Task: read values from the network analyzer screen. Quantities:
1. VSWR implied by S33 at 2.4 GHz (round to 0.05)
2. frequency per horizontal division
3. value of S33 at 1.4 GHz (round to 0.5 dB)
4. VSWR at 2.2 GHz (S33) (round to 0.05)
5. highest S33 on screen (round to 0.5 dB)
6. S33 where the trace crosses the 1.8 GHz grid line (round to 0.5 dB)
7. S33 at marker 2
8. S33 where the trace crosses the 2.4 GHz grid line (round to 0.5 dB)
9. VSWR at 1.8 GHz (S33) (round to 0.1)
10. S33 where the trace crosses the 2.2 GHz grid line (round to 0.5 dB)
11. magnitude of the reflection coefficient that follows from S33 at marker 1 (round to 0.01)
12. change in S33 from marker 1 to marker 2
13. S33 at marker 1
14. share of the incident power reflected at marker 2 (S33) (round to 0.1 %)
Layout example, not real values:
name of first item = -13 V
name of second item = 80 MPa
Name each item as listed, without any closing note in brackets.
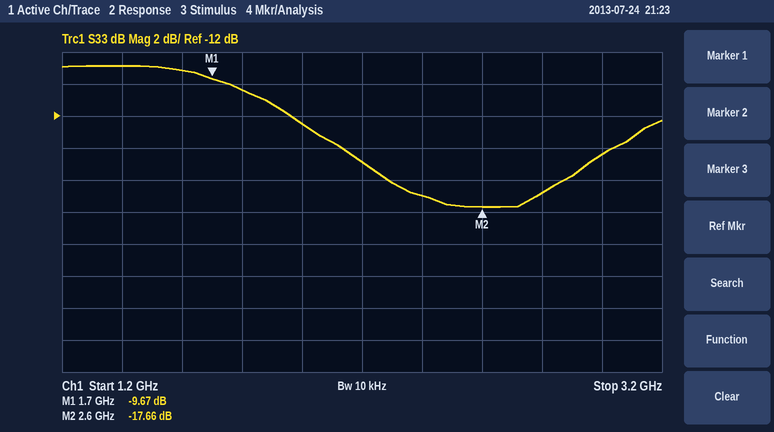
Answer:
VSWR implied by S33 at 2.4 GHz = 1.35
frequency per horizontal division = 200 MHz
value of S33 at 1.4 GHz = -9.0 dB
VSWR at 2.2 GHz (S33) = 1.45
highest S33 on screen = -9.0 dB
S33 where the trace crosses the 1.8 GHz grid line = -10.5 dB
S33 at marker 2 = -17.66 dB
S33 where the trace crosses the 2.4 GHz grid line = -17.0 dB
VSWR at 1.8 GHz (S33) = 1.9
S33 where the trace crosses the 2.2 GHz grid line = -15.0 dB
magnitude of the reflection coefficient that follows from S33 at marker 1 = 0.33
change in S33 from marker 1 to marker 2 = -7.99 dB
S33 at marker 1 = -9.67 dB
share of the incident power reflected at marker 2 (S33) = 1.7 %
